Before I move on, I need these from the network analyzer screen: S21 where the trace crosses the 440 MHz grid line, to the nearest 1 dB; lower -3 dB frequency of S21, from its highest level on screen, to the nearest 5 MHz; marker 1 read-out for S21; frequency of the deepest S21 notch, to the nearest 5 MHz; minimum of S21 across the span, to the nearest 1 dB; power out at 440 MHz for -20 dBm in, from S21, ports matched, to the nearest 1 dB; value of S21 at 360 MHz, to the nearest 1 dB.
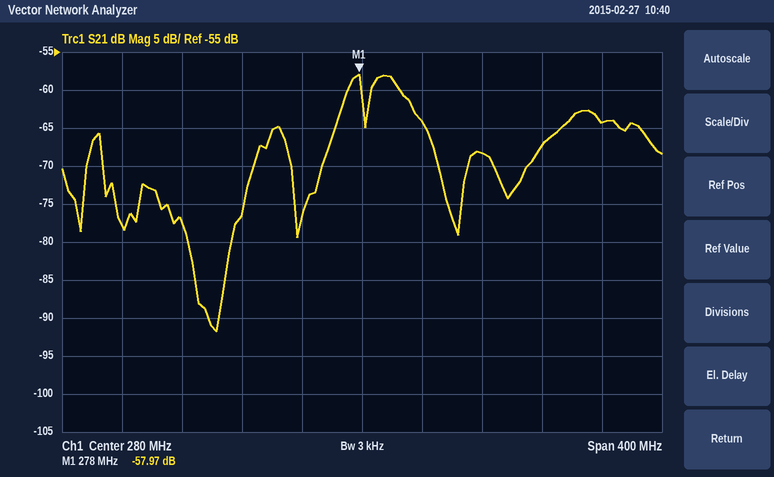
-64 dB
270 MHz
-57.97 dB
185 MHz
-92 dB
-84 dBm
-68 dB
